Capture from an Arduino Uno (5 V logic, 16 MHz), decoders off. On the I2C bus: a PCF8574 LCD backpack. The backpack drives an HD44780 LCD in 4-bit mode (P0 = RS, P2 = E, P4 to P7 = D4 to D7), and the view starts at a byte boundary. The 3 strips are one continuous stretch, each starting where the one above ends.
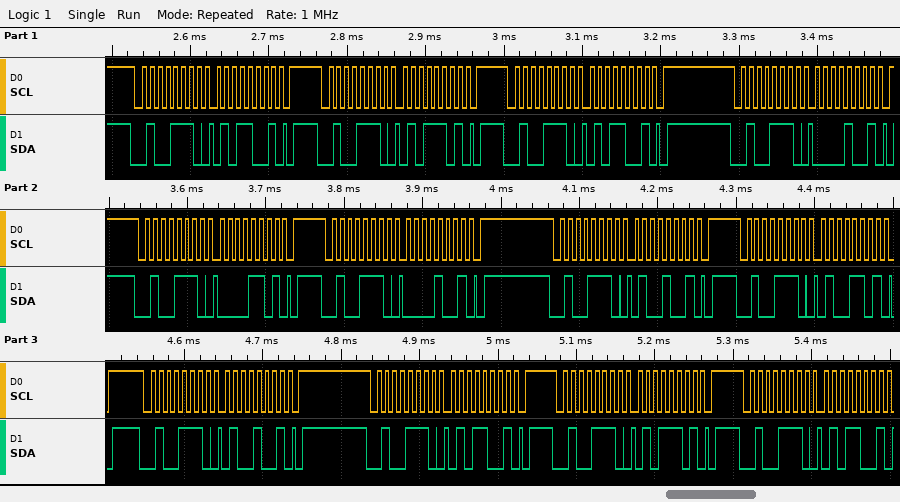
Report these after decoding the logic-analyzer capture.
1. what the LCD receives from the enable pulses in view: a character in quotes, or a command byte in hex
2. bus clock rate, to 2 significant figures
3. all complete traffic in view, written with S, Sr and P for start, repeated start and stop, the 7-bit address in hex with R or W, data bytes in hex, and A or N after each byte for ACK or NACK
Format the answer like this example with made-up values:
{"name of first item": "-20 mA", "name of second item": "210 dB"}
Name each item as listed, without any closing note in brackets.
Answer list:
{"what the LCD receives from the enable pulses in view: a character in quotes, or a command byte in hex": "'P' 'E'", "bus clock rate, to 2 significant figures": "100 kHz", "all complete traffic in view, written with S, Sr and P for start, repeated start and stop, the 7-bit address in hex with R or W, data bytes in hex, and A or N after each byte for ACK or NACK": "S 27W A 59 A P S 27W A 5D A P S 27W A 59 A P S 27W A 09 A P S 27W A 0D A P S 27W A 09 A P S 27W A 49 A P S 27W A 4D A P S 27W A 49 A P S 27W A 59 A P S 27W A 5D A P S 27W A 59 A"}
